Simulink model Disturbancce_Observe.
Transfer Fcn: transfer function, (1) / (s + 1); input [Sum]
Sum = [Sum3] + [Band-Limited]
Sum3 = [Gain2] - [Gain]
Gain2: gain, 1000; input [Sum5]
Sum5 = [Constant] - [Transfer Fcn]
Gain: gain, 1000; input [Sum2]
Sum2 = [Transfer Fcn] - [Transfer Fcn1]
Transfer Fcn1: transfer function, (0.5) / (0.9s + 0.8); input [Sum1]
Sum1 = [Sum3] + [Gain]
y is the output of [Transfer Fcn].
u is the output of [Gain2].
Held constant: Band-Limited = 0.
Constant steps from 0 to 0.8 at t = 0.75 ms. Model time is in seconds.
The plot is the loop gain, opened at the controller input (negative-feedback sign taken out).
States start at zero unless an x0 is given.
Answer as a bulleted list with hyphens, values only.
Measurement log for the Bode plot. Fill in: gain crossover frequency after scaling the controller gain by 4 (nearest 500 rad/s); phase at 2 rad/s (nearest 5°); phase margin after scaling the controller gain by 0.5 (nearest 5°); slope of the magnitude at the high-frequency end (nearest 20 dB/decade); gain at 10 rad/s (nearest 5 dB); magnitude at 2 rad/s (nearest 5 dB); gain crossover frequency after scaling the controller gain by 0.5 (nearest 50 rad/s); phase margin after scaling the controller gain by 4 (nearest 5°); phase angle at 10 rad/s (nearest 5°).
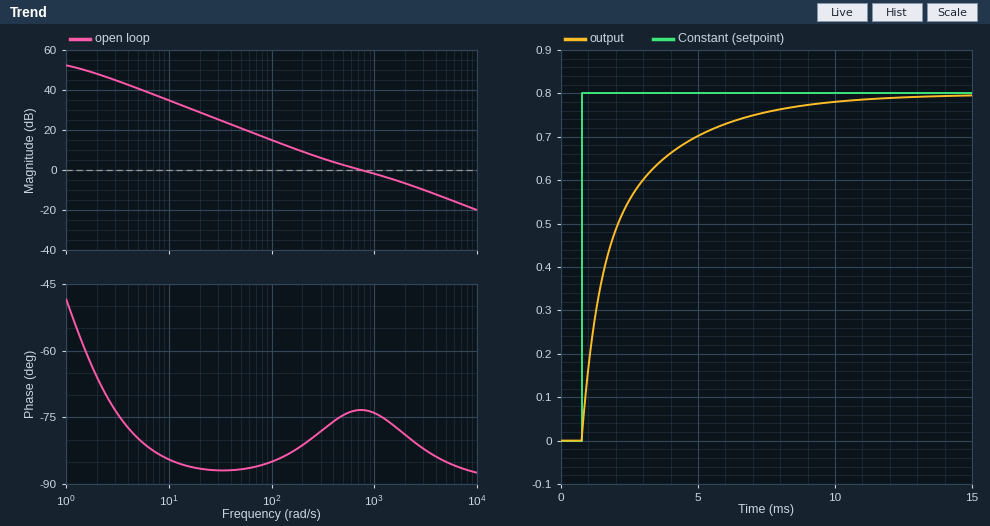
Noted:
- 4000 rad/s
- -65°
- 100°
- -20 dB/decade
- 35 dB
- 50 dB
- 300 rad/s
- 95°
- -85°
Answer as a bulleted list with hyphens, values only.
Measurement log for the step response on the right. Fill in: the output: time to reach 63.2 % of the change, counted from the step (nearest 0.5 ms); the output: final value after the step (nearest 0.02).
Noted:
- 1.5 ms
- 0.80
